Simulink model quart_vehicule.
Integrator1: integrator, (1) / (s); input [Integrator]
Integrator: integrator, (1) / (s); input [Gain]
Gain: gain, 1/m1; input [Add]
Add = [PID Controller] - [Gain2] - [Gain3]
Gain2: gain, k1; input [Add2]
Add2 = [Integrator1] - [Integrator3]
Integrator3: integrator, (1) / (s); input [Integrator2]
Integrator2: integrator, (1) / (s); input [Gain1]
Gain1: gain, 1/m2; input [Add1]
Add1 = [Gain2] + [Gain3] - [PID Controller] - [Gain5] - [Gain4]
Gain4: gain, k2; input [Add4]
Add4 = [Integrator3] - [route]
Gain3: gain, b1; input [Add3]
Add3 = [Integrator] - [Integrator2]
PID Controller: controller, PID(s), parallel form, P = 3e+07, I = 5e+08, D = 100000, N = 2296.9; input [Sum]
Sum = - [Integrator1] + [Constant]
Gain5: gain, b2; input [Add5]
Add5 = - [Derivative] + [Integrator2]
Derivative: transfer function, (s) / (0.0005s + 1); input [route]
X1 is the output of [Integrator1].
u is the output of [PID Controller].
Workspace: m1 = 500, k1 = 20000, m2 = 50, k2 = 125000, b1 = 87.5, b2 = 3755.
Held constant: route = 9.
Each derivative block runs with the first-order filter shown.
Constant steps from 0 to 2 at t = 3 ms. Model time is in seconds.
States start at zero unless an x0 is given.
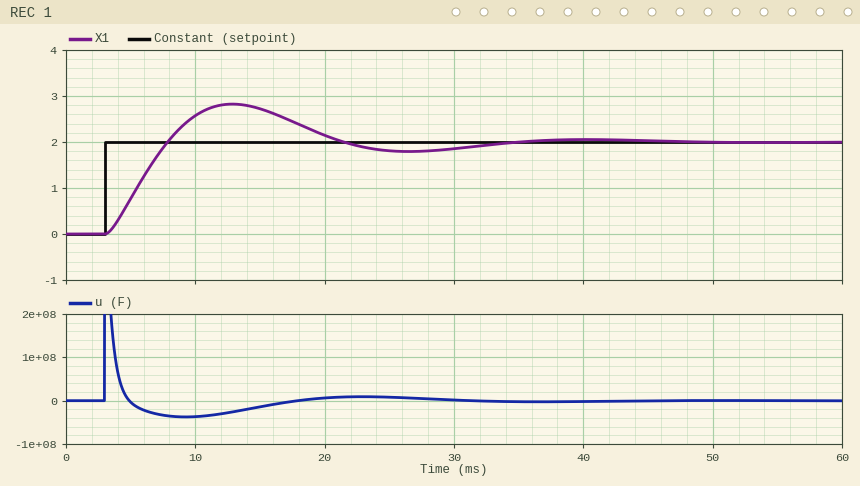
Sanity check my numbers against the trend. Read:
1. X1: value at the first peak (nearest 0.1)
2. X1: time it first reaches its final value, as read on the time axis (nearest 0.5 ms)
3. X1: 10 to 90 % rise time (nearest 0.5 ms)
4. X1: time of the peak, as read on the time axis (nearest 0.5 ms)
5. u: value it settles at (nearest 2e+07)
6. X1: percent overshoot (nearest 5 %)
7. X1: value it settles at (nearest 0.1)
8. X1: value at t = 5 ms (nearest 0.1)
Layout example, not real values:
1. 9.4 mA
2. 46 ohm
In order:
1. 2.8
2. 8.0 ms
3. 3.5 ms
4. 13.0 ms
5. 0
6. 40 %
7. 2.0
8. 0.8
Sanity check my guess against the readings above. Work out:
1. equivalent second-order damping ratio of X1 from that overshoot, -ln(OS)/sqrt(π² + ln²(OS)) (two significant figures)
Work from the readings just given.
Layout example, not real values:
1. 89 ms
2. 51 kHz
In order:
1. 0.28
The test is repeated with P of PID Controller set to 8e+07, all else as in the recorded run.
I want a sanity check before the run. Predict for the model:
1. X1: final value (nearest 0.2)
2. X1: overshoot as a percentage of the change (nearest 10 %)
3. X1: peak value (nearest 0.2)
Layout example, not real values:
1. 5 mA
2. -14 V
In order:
1. 2.0
2. 60 %
3. 3.2
